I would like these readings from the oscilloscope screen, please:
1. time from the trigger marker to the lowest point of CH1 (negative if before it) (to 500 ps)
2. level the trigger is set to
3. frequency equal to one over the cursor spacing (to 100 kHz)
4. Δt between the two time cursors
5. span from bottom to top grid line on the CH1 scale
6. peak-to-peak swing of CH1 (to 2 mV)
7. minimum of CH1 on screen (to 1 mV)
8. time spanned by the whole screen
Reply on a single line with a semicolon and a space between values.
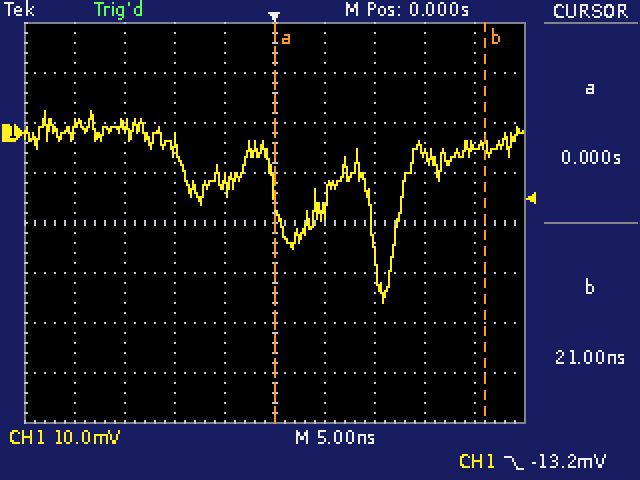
+11.0 ns; -13.2 mV; 47.6 MHz; 21.0 ns; 80 mV; 38 mV; -34 mV; 50 ns
